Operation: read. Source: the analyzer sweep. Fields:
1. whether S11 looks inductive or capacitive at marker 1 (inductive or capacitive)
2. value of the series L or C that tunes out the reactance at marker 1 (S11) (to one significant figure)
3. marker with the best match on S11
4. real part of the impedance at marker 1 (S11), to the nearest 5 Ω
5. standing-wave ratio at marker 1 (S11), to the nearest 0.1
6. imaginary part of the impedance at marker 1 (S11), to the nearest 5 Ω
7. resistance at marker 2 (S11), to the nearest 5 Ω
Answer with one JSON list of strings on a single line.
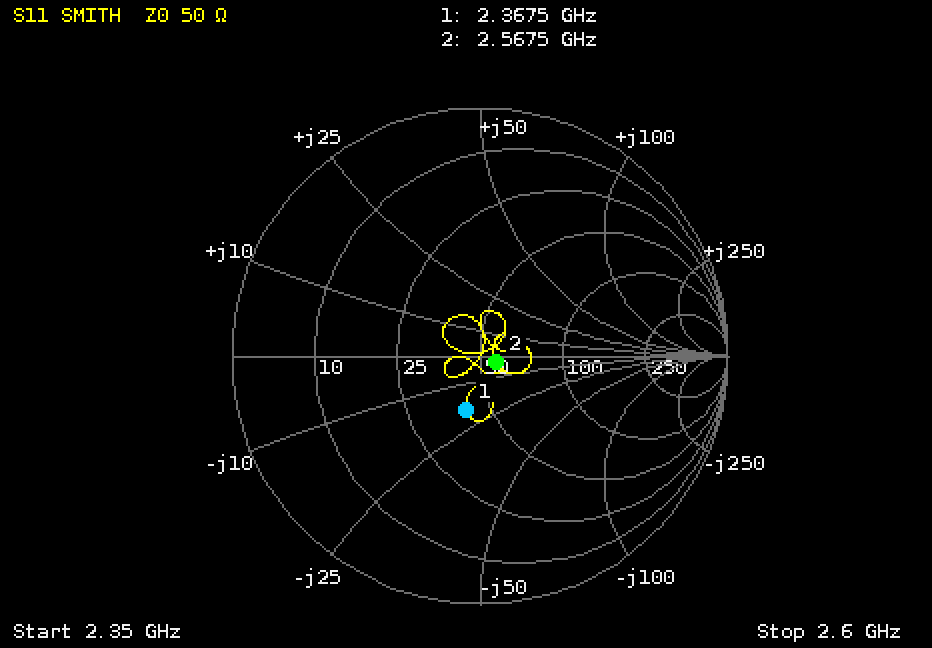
["capacitive", "1 nH", "marker 2", "40 Ω", "1.6", "-20 Ω", "55 Ω"]
